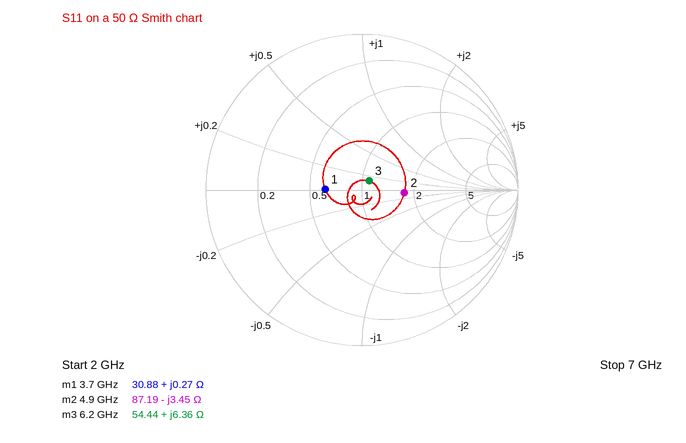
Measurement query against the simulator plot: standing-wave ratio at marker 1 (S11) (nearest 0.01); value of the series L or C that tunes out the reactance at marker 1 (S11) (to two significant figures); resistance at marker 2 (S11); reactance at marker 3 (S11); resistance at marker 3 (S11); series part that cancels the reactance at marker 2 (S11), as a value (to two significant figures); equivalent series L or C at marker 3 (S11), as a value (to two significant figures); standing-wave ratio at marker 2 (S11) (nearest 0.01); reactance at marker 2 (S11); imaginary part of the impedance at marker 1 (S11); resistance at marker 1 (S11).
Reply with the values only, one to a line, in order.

1.62
160 pF
87.19 Ω
+6.36 Ω
54.44 Ω
110 pH
160 pH
1.75
-3.45 Ω
+0.27 Ω
30.88 Ω
